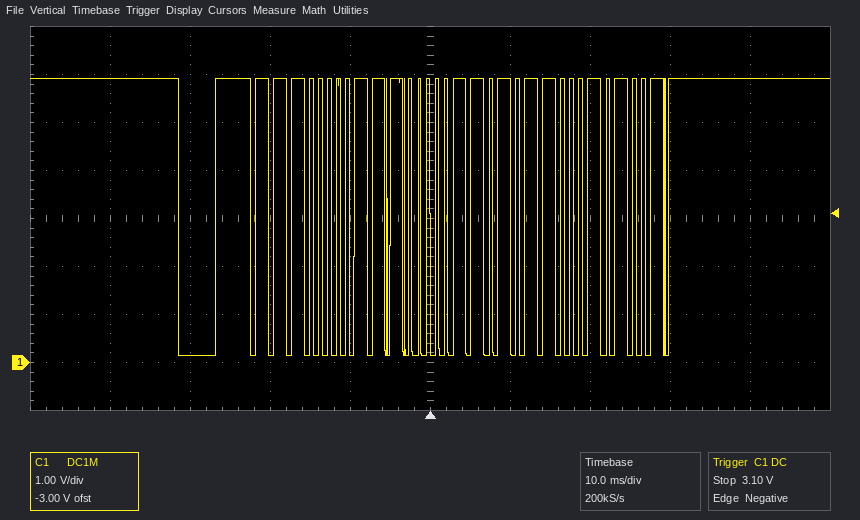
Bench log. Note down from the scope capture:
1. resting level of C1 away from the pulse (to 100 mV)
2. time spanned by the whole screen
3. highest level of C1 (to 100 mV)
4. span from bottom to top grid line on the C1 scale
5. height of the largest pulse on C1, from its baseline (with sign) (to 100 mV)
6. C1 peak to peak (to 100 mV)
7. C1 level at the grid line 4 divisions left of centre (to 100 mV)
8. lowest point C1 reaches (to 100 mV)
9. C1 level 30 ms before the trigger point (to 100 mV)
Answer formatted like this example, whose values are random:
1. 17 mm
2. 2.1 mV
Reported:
1. 5.9 V
2. 100 ms
3. 5.9 V
4. 8 V
5. -5.8 V
6. 5.8 V
7. 5.9 V
8. 100 mV
9. 100 mV
